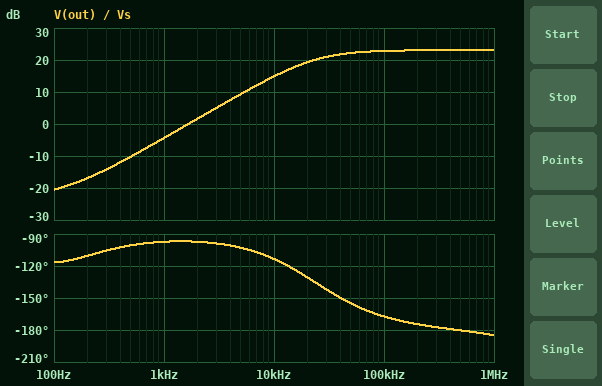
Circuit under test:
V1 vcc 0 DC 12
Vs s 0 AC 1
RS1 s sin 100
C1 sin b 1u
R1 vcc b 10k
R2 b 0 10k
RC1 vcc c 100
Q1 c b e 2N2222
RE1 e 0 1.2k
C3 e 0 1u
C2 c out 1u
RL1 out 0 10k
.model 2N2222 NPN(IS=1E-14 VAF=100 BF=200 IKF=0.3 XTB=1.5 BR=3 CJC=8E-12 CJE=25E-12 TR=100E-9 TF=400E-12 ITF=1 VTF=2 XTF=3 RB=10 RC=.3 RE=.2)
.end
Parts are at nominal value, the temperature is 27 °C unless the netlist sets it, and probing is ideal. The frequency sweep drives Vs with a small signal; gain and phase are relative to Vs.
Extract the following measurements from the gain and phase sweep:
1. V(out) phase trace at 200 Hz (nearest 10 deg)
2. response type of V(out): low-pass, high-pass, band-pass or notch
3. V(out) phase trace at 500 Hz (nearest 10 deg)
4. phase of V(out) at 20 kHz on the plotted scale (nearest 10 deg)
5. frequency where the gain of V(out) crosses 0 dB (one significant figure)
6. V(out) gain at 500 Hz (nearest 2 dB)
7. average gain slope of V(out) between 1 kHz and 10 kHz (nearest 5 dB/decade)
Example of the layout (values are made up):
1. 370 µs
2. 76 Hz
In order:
1. -110 deg
2. high-pass
3. -100 deg
4. -130 deg
5. 2 kHz
6. -10 dB
7. 20 dB/decade
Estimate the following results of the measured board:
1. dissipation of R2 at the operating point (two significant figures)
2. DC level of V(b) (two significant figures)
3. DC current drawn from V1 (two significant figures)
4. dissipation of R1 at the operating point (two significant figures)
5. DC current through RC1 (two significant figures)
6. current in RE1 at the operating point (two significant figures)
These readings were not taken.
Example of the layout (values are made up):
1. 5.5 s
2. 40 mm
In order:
1. 3.5 mW
2. 5.9 V
3. 4.9 mA
4. 3.7 mW
5. 4.3 mA
6. 4.3 mA
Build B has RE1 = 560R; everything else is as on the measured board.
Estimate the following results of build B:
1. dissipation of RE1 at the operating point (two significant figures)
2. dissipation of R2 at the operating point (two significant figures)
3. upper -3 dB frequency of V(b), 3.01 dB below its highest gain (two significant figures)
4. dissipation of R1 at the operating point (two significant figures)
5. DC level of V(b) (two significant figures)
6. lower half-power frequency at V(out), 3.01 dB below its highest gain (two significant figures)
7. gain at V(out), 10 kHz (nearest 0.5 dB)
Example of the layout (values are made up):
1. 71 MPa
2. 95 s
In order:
1. 46 mW
2. 3.3 mW
3. 4.3 MHz
4. 3.9 mW
5. 5.8 V
6. 43 kHz
7. 15.5 dB
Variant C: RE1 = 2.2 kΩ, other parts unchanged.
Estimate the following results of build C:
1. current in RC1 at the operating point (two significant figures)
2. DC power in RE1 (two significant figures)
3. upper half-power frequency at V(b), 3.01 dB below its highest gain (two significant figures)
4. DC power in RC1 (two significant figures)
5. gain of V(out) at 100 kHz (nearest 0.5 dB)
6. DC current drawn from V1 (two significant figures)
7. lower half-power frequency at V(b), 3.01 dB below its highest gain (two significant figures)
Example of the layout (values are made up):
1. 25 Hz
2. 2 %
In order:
1. 2.4 mA
2. 13 mW
3. 13 MHz
4. 570 µW
5. 18.5 dB
6. 3.0 mA
7. 31 Hz
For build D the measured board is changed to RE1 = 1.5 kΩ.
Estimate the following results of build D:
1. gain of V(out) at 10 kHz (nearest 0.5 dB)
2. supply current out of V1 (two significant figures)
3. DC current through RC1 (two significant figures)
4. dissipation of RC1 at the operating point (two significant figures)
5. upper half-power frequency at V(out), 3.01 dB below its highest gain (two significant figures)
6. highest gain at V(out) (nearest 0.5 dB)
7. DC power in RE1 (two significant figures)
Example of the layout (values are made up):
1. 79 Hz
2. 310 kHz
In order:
1. 14.5 dB
2. 4.1 mA
3. 3.5 mA
4. 1.2 mW
5. 11 MHz
6. 21.5 dB
7. 18 mW
